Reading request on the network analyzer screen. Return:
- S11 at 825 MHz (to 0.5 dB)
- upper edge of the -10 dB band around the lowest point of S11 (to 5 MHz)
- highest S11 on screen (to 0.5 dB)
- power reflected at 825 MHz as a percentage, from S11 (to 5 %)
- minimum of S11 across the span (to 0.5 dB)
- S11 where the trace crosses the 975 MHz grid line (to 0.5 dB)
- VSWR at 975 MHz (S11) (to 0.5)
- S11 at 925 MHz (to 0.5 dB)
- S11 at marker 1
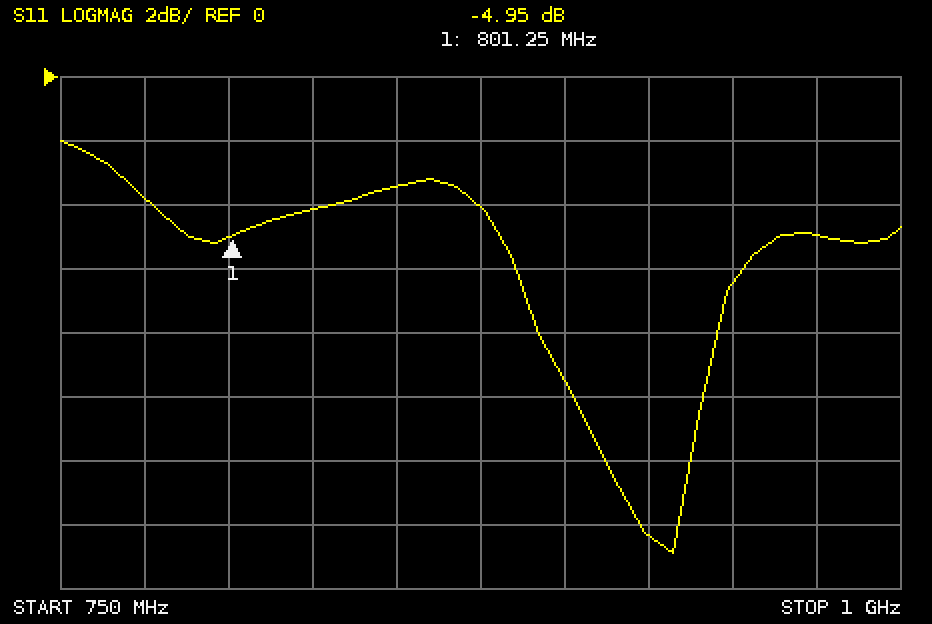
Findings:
-4.0 dB
940 MHz
-2.0 dB
40 %
-15.0 dB
-5.0 dB
3.5
-14.5 dB
-4.95 dB
